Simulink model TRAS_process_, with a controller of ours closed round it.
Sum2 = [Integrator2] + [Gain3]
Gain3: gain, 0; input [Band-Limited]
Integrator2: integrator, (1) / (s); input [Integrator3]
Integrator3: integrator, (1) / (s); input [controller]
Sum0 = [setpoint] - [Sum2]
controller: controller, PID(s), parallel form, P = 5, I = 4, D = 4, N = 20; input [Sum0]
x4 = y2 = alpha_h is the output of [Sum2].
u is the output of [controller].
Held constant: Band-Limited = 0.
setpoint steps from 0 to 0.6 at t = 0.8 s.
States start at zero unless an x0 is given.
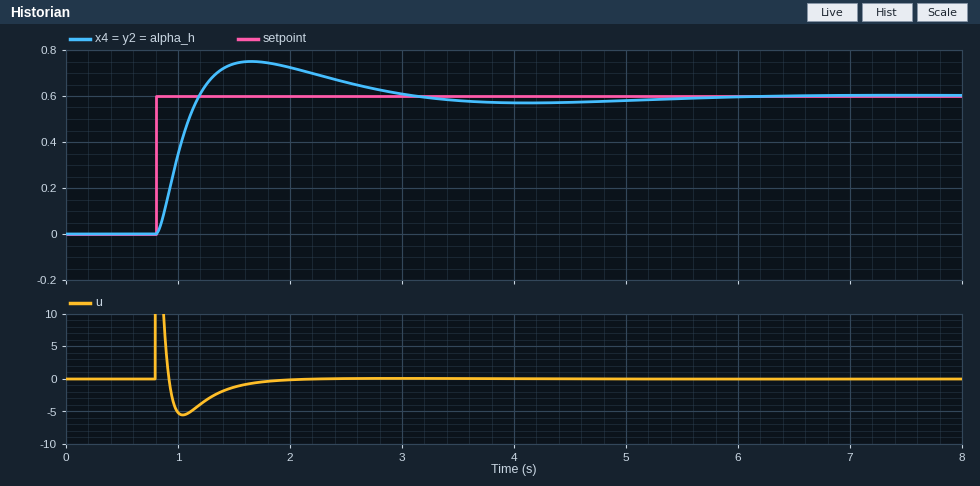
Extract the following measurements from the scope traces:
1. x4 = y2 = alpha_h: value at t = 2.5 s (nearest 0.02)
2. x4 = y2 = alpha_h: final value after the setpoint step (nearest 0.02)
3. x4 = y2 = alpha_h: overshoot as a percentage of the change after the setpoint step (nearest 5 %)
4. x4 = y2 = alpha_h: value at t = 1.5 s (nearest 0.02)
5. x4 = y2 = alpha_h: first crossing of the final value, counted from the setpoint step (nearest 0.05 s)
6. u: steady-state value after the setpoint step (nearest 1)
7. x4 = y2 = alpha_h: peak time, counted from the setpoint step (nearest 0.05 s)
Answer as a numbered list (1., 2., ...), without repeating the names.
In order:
1. 0.66
2. 0.60
3. 25 %
4. 0.74
5. 0.40 s
6. 0
7. 0.85 s
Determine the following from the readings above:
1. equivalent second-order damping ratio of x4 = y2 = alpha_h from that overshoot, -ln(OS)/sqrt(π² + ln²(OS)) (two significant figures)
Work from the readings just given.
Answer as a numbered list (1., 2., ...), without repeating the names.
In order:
1. 0.40
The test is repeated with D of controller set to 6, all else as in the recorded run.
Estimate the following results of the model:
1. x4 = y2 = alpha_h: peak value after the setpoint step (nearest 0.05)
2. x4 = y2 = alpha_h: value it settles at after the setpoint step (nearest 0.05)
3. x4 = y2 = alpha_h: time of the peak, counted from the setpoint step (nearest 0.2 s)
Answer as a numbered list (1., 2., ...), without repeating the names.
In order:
1. 0.70
2. 0.60
3. 0.6 s
